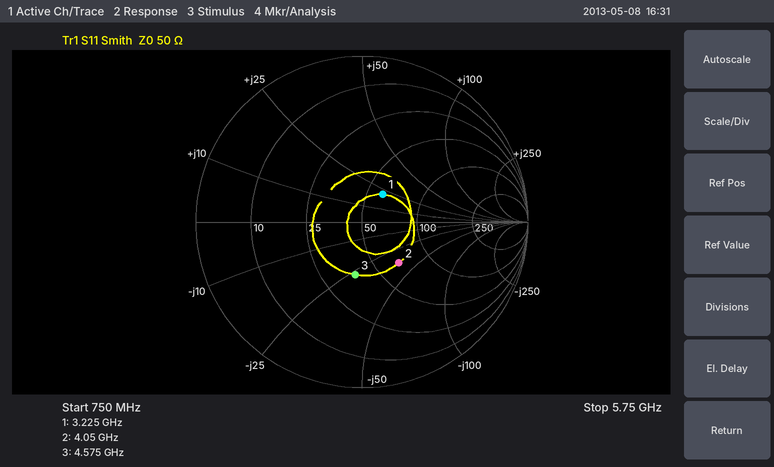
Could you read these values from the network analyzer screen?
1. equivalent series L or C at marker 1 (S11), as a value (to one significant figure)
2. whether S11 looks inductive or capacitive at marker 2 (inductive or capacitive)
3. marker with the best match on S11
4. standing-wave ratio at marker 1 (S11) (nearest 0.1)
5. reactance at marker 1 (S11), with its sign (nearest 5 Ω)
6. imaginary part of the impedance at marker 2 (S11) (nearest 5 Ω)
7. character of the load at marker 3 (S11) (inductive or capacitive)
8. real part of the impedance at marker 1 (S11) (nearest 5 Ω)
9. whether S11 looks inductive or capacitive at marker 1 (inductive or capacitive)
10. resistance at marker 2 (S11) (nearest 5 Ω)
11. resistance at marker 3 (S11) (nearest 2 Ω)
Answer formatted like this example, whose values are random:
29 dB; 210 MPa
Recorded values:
1 nH; capacitive; marker 1; 1.5; +20 Ω; -35 Ω; capacitive; 60 Ω; inductive; 65 Ω; 38 Ω
